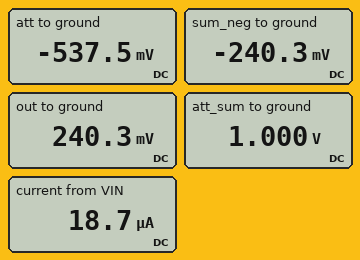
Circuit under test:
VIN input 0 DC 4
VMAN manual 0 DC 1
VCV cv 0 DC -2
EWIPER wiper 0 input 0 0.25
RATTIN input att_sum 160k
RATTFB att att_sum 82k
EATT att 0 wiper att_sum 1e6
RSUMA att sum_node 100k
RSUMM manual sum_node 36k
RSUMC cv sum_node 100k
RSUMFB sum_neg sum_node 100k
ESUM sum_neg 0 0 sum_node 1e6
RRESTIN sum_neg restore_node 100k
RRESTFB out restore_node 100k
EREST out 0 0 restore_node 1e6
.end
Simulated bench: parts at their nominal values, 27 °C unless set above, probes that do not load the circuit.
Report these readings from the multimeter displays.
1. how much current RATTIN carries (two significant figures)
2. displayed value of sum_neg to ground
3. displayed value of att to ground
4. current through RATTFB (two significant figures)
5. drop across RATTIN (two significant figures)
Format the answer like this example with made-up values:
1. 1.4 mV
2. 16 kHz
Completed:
1. 19 µA
2. -240.3 mV
3. -537.5 mV
4. 19 µA
5. 3.0 V
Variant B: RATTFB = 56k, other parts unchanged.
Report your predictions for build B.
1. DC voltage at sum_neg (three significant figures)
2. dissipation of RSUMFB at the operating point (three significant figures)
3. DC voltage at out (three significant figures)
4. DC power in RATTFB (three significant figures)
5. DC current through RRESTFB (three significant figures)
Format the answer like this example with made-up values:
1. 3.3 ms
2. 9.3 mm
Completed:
1. -728 mV
2. 5.30 µW
3. 728 mV
4. 19.7 µW
5. 7.28 µA
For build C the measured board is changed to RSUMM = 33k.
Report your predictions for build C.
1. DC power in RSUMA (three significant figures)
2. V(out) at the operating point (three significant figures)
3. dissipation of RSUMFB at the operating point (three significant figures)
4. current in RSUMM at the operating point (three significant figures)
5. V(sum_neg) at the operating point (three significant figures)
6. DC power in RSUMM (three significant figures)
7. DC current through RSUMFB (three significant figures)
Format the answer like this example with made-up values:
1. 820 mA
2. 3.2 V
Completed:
1. 2.89 µW
2. 493 mV
3. 2.43 µW
4. 30.3 µA
5. -493 mV
6. 30.3 µW
7. 4.93 µA
